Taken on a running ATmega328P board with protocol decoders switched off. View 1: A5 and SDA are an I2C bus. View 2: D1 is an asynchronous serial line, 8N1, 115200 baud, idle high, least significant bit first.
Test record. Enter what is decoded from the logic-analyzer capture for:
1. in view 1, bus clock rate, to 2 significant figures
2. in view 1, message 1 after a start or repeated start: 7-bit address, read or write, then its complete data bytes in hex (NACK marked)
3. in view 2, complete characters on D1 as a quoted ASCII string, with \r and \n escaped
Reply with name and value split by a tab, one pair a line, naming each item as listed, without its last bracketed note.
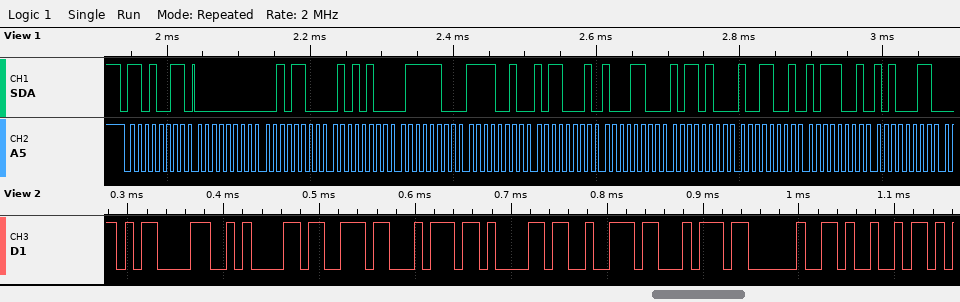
in view 1, bus clock rate, to 2 significant figures	100 kHz
in view 1, message 1 after a start or repeated start: 7-bit address, read or write, then its complete data bytes in hex	0x69 read: 00 2C 54 7C F2 B1 8C B4 99 B9 A3
in view 2, complete characters on D1 as a quoted ASCII string, with \r and \n escaped	"\r\nstart I"
